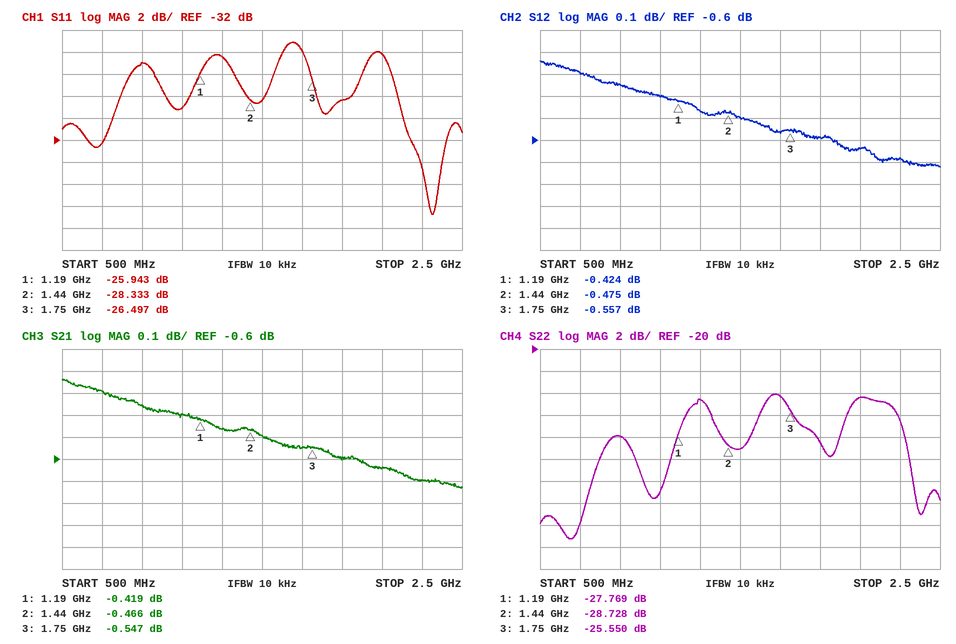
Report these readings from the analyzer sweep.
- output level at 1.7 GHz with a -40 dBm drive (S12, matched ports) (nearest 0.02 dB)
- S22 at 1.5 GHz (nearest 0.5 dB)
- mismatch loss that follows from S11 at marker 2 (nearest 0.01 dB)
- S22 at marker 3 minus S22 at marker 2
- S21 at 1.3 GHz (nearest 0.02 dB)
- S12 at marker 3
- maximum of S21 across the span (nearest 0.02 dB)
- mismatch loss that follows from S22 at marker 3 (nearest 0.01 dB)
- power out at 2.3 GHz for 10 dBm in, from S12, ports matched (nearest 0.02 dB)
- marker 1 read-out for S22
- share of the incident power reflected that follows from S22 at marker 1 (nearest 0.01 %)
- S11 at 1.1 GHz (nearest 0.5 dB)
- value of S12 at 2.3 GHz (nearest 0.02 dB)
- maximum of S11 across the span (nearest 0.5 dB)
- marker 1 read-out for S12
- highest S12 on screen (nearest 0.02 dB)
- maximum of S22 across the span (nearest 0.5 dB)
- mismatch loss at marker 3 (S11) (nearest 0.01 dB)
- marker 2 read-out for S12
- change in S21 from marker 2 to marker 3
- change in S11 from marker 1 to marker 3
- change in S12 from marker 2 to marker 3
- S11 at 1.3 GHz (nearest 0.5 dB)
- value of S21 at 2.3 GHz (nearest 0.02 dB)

-40.56 dBm
-29.0 dB
0.01 dB
3.178 dB
-0.46 dB
-0.557 dB
-0.24 dB
0.01 dB
9.32 dBm
-27.769 dB
0.17 %
-29.0 dB
-0.68 dB
-23.0 dB
-0.424 dB
-0.24 dB
-24.0 dB
0.01 dB
-0.475 dB
-0.081 dB
-0.554 dB
-0.082 dB
-24.5 dB
-0.70 dB
